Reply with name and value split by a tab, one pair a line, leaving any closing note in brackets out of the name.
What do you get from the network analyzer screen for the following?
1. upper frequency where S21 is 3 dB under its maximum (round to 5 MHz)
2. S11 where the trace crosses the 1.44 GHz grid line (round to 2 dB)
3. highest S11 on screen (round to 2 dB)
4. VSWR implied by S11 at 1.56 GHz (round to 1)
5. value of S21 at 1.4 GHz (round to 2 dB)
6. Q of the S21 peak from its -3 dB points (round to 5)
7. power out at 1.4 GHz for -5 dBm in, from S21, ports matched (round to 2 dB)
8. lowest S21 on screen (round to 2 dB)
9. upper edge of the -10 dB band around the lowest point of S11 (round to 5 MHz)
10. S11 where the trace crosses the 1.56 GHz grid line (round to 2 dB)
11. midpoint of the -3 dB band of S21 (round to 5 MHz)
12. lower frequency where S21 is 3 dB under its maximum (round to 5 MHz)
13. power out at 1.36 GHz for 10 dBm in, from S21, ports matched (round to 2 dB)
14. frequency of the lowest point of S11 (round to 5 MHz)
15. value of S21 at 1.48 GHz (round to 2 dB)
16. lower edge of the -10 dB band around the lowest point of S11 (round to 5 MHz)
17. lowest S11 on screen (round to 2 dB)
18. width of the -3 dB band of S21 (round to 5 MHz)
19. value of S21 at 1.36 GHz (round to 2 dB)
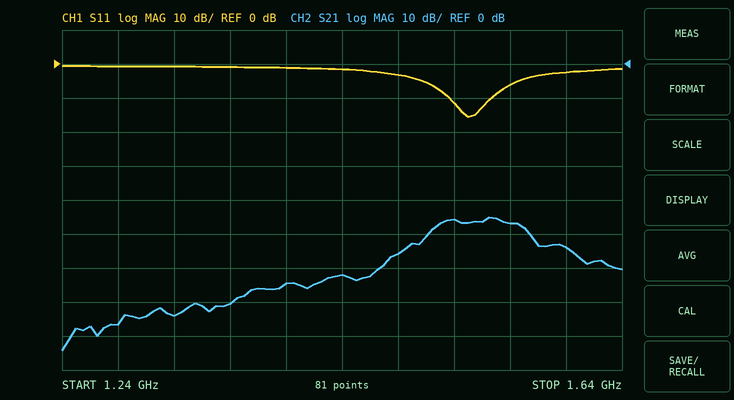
upper frequency where S21 is 3 dB under its maximum	1.570 GHz
S11 where the trace crosses the 1.44 GHz grid line	-2 dB
highest S11 on screen	0 dB
VSWR implied by S11 at 1.56 GHz	3
value of S21 at 1.4 GHz	-64 dB
Q of the S21 peak from its -3 dB points	25
power out at 1.4 GHz for -5 dBm in, from S21, ports matched	-70 dBm
lowest S21 on screen	-84 dB
upper edge of the -10 dB band around the lowest point of S11	1.545 GHz
S11 where the trace crosses the 1.56 GHz grid line	-6 dB
midpoint of the -3 dB band of S21	1.540 GHz
lower frequency where S21 is 3 dB under its maximum	1.505 GHz
power out at 1.36 GHz for 10 dBm in, from S21, ports matched	-60 dBm
frequency of the lowest point of S11	1.530 GHz
value of S21 at 1.48 GHz	-56 dB
lower edge of the -10 dB band around the lowest point of S11	1.515 GHz
lowest S11 on screen	-16 dB
width of the -3 dB band of S21	65 MHz
value of S21 at 1.36 GHz	-70 dB
